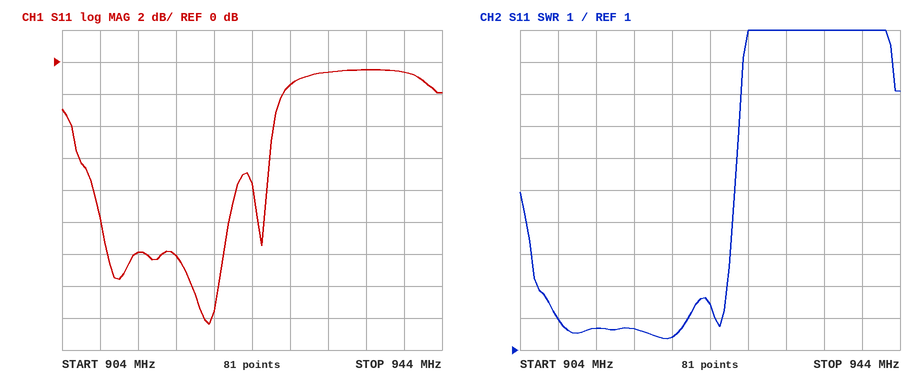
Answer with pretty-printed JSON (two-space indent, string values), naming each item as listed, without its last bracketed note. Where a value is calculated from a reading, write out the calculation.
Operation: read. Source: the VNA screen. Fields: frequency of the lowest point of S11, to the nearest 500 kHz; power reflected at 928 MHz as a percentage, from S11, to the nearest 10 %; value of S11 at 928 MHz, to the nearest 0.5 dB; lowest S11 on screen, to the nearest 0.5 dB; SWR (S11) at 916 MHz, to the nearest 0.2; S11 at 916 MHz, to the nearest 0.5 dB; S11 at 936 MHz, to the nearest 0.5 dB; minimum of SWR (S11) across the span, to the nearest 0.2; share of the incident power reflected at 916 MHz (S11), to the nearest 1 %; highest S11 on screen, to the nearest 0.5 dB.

{
  "frequency of the lowest point of S11, to the nearest 500 kHz": "919.5 MHz",
  "power reflected at 928 MHz as a percentage, from S11, to the nearest 10 %": "10^(-1.5/10) ≈ 70.8 %, so 70 % to the nearest 10 %",
  "value of S11 at 928 MHz, to the nearest 0.5 dB": "-1.5 dB",
  "lowest S11 on screen, to the nearest 0.5 dB": "-16.5 dB",
  "SWR (S11) at 916 MHz, to the nearest 0.2": "1.6",
  "S11 at 916 MHz, to the nearest 0.5 dB": "-12.0 dB",
  "S11 at 936 MHz, to the nearest 0.5 dB": "-0.5 dB",
  "minimum of SWR (S11) across the span, to the nearest 0.2": "1.4",
  "share of the incident power reflected at 916 MHz (S11), to the nearest 1 %": "10^(-12/10) ≈ 6 %",
  "highest S11 on screen, to the nearest 0.5 dB": "-0.5 dB"
}
